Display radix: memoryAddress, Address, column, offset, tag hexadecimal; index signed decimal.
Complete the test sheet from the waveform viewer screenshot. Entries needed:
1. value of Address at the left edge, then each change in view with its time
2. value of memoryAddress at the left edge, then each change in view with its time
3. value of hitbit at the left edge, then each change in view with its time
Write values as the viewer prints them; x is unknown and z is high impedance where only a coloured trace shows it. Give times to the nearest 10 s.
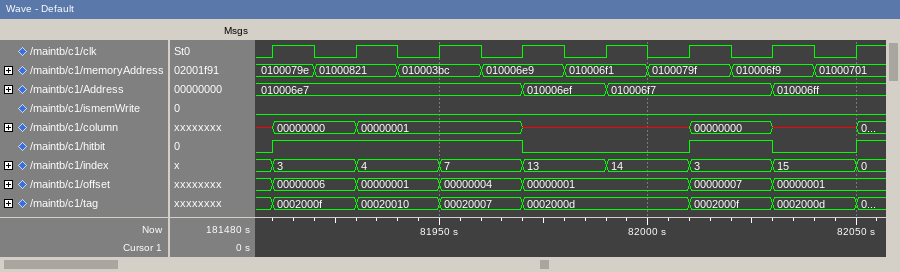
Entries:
010006e7, 010006ef at 81970 s, 010006f7 at 81990 s, 010006ff at 82030 s
0100079e, 01000821 at 81920 s, 010003bc at 81940 s, 010006e9 at 81960 s, 010006f1 at 81980 s, 0100079f at 82000 s, 010006f9 at 82020 s, 01000701 at 82040 s
0, 1 at 81910 s, 0 at 81970 s, 1 at 82010 s, 0 at 82030 s, 1 at 82050 s
